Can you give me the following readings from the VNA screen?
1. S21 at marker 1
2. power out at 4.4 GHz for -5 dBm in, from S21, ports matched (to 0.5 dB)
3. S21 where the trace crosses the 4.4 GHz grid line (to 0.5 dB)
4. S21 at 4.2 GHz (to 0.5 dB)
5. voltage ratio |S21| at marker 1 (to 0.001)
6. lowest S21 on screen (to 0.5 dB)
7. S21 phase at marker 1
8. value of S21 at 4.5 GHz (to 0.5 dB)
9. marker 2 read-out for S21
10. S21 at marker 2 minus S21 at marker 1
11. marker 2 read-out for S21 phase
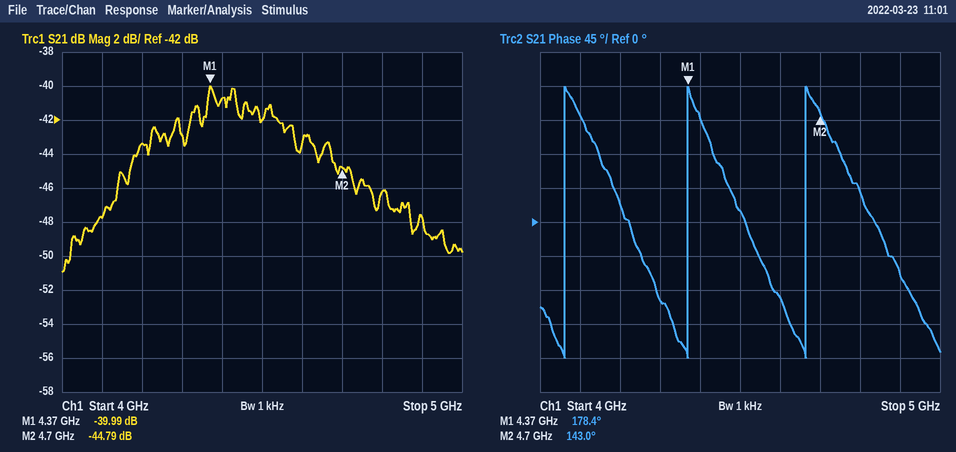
-39.99 dB
-45.5 dBm
-40.5 dB
-43.5 dB
0.010
-51.0 dB
178.4°
-42.0 dB
-44.79 dB
-4.80 dB
143.0°
